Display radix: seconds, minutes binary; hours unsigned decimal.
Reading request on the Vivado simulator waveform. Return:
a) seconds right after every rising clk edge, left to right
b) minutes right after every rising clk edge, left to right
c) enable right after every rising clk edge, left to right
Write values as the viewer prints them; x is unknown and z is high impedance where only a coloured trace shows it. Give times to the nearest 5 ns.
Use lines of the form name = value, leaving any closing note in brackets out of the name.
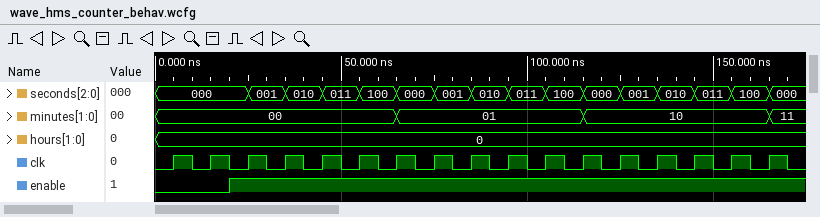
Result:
seconds right after every rising clk edge, left to right = 000, 000, 001, 010, 011, 100, 000, 001, 010, 011, 100, 000, 001, 010, 011, 100, 000
minutes right after every rising clk edge, left to right = 00, 00, 00, 00, 00, 00, 01, 01, 01, 01, 01, 10, 10, 10, 10, 10, 11
enable right after every rising clk edge, left to right = 0 0 1 1 1 1 1 1 1 1 1 1 1 1 1 1 1
